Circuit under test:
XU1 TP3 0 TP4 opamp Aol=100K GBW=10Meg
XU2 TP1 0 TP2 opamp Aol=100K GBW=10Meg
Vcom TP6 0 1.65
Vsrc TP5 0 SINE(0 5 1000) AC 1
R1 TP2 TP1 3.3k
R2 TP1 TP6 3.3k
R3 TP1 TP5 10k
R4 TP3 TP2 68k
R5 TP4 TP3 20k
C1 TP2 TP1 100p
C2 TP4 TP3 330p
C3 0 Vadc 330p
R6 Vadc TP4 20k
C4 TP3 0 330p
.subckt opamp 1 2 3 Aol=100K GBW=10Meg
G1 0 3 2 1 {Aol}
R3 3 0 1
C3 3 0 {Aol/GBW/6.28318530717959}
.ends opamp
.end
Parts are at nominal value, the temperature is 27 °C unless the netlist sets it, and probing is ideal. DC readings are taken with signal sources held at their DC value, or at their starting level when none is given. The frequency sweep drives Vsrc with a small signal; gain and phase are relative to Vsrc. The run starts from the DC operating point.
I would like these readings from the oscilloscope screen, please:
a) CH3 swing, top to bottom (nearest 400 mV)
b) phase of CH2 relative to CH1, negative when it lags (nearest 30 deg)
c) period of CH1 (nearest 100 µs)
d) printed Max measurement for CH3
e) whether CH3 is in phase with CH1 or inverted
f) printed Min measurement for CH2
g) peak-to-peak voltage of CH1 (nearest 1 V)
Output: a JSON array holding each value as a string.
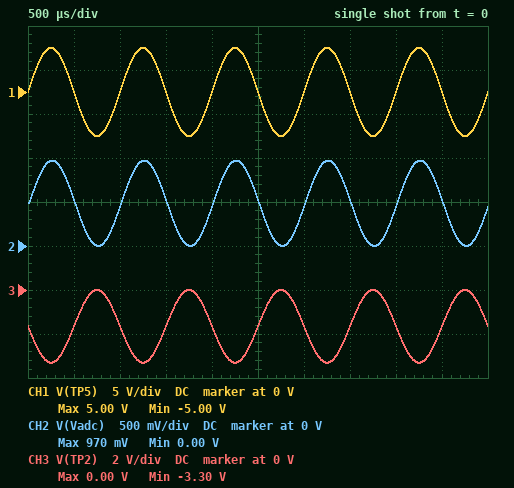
["3.2 V", "0 deg", "1.0 ms", "0.00 V", "inverted", "0.00 V", "10 V"]
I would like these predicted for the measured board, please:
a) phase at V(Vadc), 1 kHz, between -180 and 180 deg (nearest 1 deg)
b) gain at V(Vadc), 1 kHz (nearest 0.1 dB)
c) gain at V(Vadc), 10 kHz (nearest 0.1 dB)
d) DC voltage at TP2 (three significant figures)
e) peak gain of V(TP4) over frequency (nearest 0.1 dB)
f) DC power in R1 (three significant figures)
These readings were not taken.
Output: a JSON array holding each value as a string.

["-5 deg", "-20.3 dB", "-21.6 dB", "-1.65 V", "-20.3 dB", "825 µW"]
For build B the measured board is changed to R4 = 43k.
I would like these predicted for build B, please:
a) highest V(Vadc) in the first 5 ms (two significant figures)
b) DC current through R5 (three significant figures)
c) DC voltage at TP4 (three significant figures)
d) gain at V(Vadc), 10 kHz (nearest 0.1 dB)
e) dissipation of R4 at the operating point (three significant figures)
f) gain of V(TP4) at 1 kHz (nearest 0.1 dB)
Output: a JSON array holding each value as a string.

["1.5 V", "38.4 µA", "767 mV", "-17.7 dB", "63.3 µW", "-16.3 dB"]
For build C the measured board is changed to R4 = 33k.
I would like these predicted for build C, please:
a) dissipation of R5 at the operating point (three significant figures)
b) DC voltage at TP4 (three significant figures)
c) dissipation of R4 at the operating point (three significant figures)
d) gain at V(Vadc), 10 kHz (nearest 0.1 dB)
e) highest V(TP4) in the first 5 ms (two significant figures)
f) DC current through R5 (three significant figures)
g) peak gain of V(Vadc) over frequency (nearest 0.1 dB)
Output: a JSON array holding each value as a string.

["50.0 µW", "1.00 V", "82.5 µW", "-15.4 dB", "2.0 V", "50.0 µA", "-14.0 dB"]
